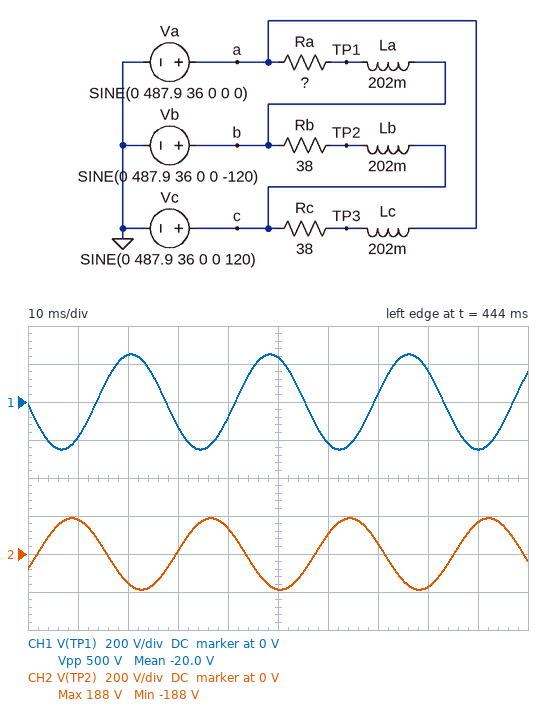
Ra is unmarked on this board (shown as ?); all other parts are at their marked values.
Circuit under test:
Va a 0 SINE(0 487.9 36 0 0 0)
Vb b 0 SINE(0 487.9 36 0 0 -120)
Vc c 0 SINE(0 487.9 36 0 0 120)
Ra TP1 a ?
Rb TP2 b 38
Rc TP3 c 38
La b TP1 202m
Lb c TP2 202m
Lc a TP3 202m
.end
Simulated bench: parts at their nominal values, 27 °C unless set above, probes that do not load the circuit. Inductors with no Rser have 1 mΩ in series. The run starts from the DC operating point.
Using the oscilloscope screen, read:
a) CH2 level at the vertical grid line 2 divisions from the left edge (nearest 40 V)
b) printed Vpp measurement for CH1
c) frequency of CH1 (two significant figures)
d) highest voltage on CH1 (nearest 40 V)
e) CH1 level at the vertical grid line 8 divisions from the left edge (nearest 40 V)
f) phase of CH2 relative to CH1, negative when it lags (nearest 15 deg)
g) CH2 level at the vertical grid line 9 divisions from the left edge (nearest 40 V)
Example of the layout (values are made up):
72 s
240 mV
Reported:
-160 V
500 V
36 Hz
240 V
160 V
150 deg
160 V
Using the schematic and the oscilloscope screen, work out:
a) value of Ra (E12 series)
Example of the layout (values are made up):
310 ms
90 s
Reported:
82 Ω
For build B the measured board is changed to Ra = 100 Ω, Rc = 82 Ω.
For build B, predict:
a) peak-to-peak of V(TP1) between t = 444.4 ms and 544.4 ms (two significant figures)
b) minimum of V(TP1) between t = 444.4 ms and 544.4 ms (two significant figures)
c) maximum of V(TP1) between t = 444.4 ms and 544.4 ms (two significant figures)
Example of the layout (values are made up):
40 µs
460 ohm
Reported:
570 V
-290 V
290 V
